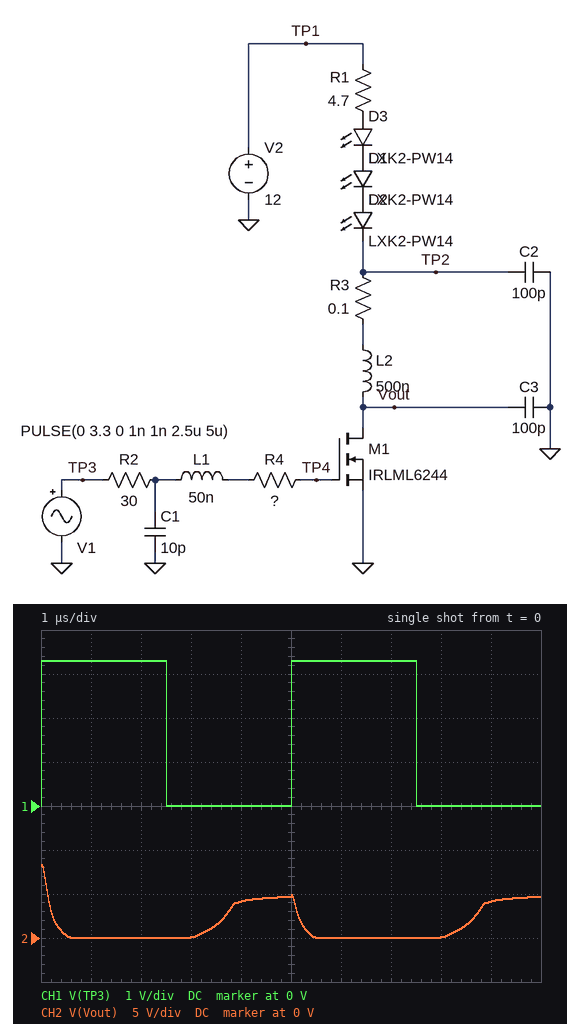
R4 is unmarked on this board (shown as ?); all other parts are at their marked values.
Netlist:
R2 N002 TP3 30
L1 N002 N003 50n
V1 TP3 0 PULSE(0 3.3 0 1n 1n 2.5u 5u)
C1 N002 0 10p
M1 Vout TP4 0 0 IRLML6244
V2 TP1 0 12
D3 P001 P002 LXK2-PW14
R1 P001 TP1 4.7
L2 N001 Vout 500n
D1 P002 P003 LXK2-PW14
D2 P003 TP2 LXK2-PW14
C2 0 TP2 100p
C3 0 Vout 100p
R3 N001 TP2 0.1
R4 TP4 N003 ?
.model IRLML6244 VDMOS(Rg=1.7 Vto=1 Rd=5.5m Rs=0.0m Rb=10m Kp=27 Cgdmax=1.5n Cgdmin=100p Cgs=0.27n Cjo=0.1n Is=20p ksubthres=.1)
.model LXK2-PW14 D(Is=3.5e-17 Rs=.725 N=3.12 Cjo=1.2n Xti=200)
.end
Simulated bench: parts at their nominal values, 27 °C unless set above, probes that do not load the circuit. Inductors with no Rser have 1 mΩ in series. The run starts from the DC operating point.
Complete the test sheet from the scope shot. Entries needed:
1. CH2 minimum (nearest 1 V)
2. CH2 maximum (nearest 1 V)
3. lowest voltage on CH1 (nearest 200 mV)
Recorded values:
0 V
8 V
0 V
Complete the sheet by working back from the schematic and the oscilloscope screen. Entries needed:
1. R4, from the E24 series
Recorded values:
270 Ω
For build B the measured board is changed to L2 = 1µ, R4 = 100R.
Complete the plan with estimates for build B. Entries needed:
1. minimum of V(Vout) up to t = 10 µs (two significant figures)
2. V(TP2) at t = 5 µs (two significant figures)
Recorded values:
9.1 mV
4.8 V
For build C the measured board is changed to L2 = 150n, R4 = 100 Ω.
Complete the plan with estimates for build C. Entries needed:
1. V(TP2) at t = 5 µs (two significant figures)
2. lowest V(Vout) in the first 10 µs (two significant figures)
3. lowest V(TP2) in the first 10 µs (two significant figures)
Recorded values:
4.8 V
9.1 mV
53 mV
